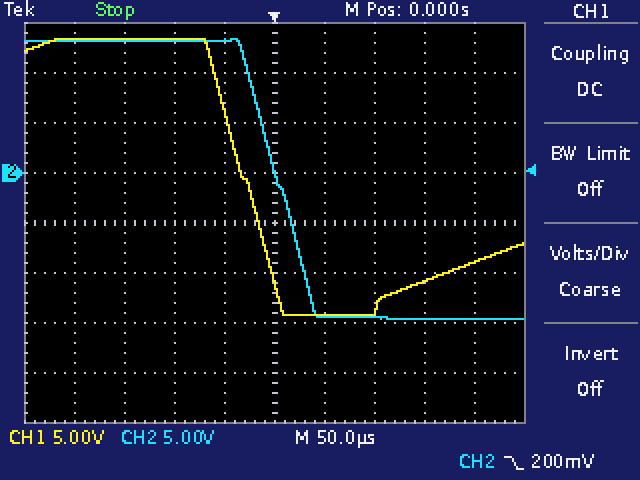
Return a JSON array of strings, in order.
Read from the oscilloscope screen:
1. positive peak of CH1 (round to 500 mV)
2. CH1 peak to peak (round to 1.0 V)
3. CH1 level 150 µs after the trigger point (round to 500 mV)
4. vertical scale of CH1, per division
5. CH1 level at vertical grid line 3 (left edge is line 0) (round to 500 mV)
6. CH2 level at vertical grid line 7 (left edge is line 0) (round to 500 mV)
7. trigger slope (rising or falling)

["13.5 V", "28.0 V", "-11.0 V", "5 V", "13.5 V", "-14.5 V", "falling"]
